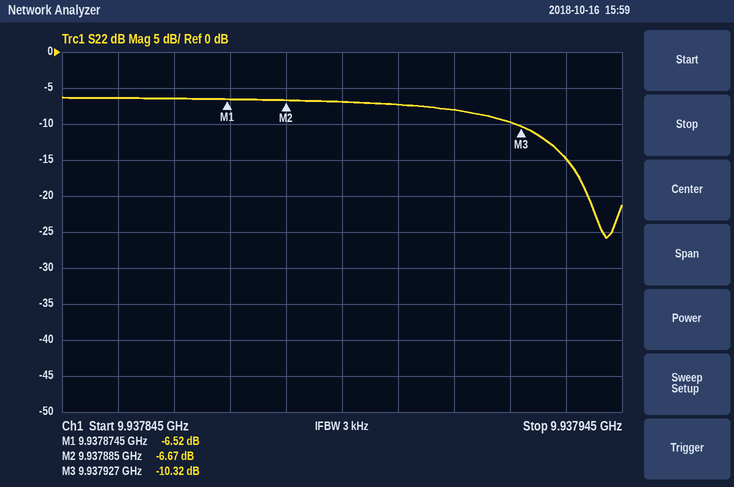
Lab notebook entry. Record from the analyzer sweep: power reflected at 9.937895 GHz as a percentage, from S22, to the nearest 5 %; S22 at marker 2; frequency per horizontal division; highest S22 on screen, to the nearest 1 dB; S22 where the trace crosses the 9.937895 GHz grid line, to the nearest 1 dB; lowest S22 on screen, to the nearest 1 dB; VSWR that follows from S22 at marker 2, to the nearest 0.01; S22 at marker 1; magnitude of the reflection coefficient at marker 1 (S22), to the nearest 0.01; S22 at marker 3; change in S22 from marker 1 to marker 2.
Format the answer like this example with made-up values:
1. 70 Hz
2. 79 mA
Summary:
1. 20 %
2. -6.67 dB
3. 10 kHz
4. -6 dB
5. -7 dB
6. -26 dB
7. 2.73
8. -6.52 dB
9. 0.47
10. -10.32 dB
11. -0.15 dB
